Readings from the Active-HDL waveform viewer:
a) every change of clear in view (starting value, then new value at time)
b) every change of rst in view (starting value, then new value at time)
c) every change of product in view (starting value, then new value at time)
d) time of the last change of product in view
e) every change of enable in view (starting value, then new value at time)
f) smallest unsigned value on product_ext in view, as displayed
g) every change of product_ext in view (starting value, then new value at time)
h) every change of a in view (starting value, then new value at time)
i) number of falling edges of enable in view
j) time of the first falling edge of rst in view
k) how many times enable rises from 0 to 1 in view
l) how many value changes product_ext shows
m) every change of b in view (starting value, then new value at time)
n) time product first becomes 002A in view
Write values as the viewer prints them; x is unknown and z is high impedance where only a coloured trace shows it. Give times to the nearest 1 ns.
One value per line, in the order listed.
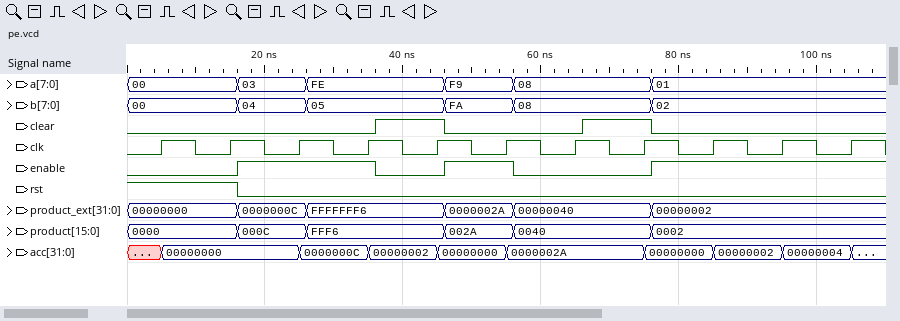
0, 1 at 36 ns, 0 at 46 ns, 1 at 66 ns, 0 at 76 ns
1, 0 at 16 ns
0000, 000C at 16 ns, FFF6 at 26 ns, 002A at 46 ns, 0040 at 56 ns, 0002 at 76 ns
76 ns
0, 1 at 16 ns, 0 at 36 ns, 1 at 46 ns, 0 at 56 ns, 1 at 76 ns
00000000
00000000, 0000000C at 16 ns, FFFFFFF6 at 26 ns, 0000002A at 46 ns, 00000040 at 56 ns, 00000002 at 76 ns
00, 03 at 16 ns, FE at 26 ns, F9 at 46 ns, 08 at 56 ns, 01 at 76 ns
2
16 ns
3
5
00, 04 at 16 ns, 05 at 26 ns, FA at 46 ns, 08 at 56 ns, 02 at 76 ns
46 ns
